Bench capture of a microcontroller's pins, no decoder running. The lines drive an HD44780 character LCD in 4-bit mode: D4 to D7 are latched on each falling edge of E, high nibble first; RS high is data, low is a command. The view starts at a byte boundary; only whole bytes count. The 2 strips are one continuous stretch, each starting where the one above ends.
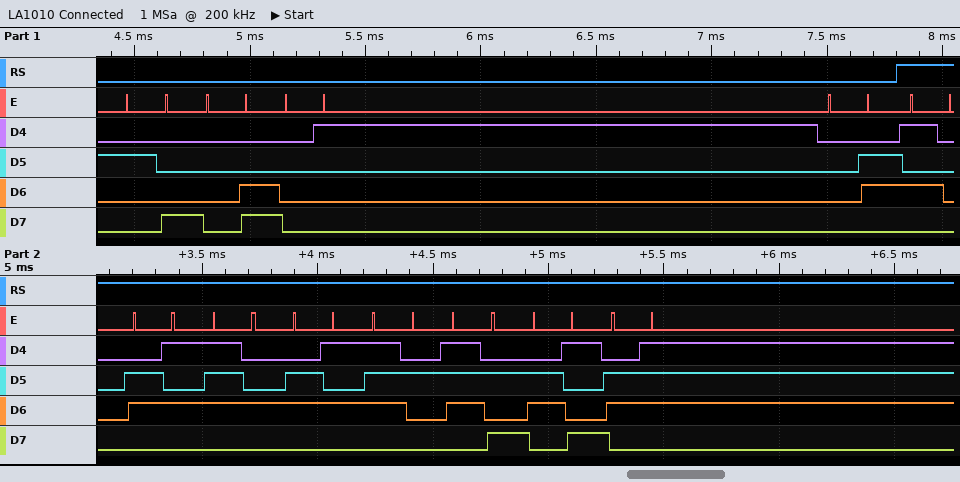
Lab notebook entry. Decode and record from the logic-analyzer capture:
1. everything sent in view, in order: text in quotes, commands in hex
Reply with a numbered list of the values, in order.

1. 0x28 0x0C 0x01 0x06 "Peterzig"
